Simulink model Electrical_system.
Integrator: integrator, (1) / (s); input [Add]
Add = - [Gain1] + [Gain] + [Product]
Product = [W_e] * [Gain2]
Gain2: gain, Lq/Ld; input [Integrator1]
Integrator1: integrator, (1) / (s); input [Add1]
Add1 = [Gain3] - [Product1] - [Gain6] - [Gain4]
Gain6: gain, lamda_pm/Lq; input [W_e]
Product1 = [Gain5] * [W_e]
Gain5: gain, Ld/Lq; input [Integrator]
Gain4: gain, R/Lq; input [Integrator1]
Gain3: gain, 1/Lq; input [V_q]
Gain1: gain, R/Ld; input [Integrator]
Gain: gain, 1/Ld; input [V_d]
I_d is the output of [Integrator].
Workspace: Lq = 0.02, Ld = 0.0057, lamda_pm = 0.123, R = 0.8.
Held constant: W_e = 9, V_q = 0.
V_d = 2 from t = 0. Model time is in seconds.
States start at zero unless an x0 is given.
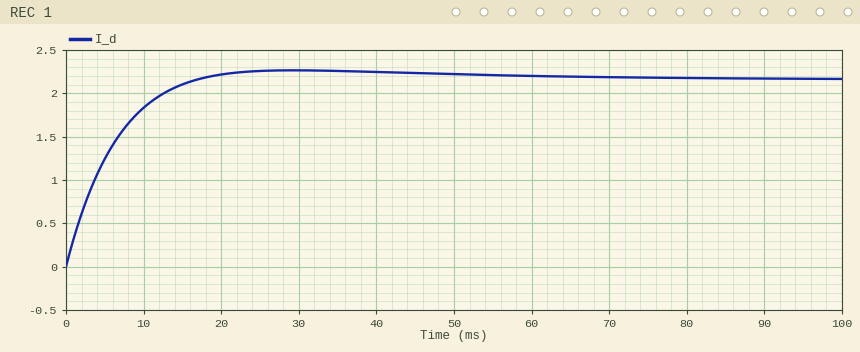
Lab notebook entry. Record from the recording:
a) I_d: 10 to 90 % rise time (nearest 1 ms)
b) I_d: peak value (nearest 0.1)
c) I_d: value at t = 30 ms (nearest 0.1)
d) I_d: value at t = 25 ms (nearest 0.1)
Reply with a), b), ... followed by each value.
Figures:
a) 11 ms
b) 2.3
c) 2.3
d) 2.3
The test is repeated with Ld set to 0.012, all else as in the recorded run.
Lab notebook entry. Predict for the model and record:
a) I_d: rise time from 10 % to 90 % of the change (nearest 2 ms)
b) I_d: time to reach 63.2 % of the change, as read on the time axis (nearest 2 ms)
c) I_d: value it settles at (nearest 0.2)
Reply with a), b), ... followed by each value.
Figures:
a) 24 ms
b) 12 ms
c) 2.2
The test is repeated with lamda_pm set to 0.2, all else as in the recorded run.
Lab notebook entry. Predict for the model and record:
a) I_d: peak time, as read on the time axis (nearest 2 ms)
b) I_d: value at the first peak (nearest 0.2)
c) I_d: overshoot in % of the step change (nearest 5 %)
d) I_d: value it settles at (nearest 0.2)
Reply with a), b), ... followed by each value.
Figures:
a) 26 ms
b) 2.2
c) 10 %
d) 2.0
